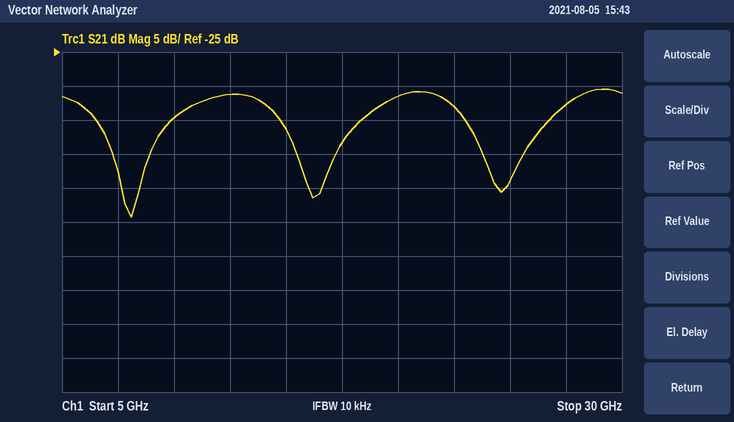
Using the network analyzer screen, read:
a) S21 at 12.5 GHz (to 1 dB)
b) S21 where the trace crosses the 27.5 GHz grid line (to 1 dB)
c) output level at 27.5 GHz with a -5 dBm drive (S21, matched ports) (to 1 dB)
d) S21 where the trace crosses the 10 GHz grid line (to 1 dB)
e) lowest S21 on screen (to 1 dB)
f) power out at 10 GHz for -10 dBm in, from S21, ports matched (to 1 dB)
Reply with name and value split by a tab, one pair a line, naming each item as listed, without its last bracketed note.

S21 at 12.5 GHz	-31 dB
S21 where the trace crosses the 27.5 GHz grid line	-33 dB
output level at 27.5 GHz with a -5 dBm drive (S21, matched ports)	-38 dBm
S21 where the trace crosses the 10 GHz grid line	-35 dB
lowest S21 on screen	-49 dB
power out at 10 GHz for -10 dBm in, from S21, ports matched	-45 dBm
